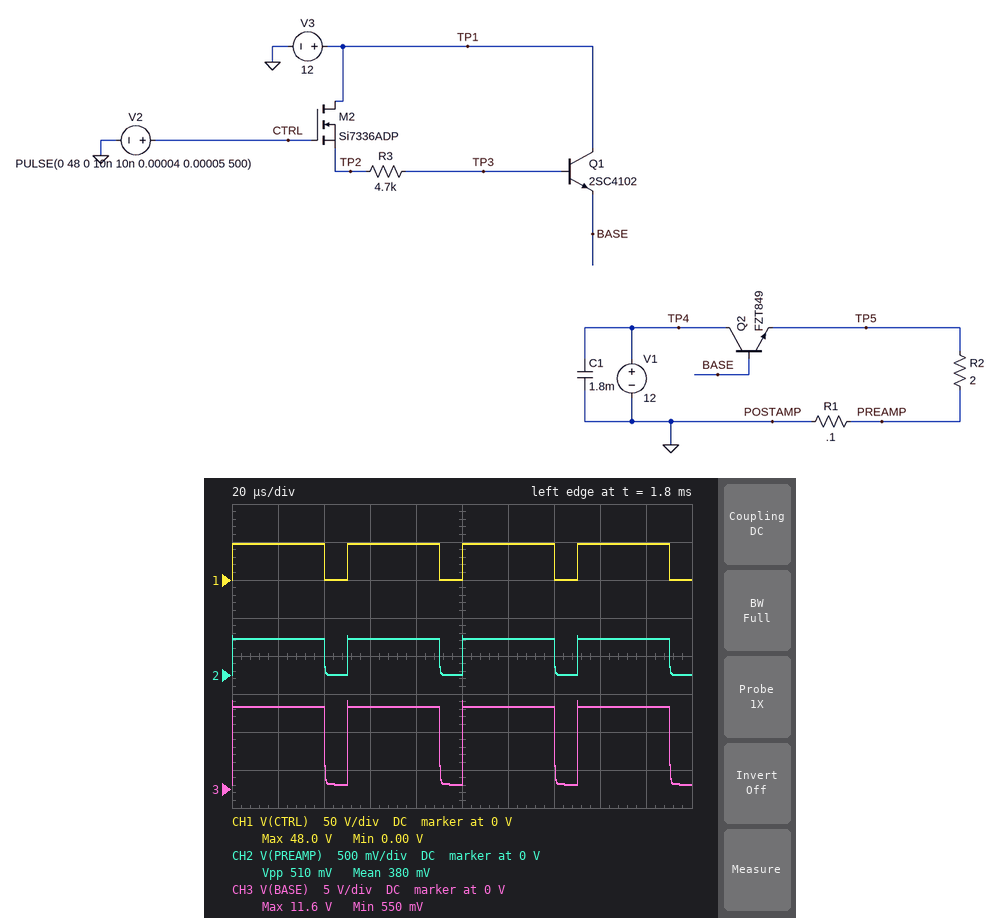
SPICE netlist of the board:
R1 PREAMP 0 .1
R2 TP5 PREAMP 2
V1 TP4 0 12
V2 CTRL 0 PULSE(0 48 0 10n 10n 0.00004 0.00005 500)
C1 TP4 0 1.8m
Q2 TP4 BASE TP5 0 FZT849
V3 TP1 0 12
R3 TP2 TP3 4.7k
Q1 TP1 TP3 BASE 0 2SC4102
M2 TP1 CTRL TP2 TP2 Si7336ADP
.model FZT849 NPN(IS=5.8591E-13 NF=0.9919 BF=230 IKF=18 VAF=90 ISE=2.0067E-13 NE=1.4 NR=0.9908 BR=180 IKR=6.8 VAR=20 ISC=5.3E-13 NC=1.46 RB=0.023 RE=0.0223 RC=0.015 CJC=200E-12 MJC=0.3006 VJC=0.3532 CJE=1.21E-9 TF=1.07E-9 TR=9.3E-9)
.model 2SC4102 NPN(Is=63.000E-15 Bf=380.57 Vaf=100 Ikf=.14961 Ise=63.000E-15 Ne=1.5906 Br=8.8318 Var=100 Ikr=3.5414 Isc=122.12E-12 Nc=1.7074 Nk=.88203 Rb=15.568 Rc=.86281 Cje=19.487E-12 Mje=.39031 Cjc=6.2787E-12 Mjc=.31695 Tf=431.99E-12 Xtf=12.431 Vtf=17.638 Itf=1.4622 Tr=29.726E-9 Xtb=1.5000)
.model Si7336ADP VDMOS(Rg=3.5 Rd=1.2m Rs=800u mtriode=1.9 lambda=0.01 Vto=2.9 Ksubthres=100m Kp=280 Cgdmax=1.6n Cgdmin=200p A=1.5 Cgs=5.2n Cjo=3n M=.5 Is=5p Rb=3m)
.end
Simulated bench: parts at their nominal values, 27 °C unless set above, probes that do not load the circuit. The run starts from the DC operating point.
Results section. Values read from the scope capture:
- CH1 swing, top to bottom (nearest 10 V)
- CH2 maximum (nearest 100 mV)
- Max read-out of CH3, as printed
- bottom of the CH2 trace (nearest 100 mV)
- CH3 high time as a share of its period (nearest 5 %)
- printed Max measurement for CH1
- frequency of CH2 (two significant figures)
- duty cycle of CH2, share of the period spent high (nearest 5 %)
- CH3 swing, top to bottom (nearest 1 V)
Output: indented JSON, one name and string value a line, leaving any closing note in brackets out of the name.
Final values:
{
  "CH1 swing, top to bottom": "50 V",
  "CH2 maximum": "500 mV",
  "Max read-out of CH3, as printed": "11.6 V",
  "bottom of the CH2 trace": "0 V",
  "CH3 high time as a share of its period": "80 %",
  "printed Max measurement for CH1": "48.0 V",
  "frequency of CH2": "20 kHz",
  "duty cycle of CH2, share of the period spent high": "80 %",
  "CH3 swing, top to bottom": "11 V"
}
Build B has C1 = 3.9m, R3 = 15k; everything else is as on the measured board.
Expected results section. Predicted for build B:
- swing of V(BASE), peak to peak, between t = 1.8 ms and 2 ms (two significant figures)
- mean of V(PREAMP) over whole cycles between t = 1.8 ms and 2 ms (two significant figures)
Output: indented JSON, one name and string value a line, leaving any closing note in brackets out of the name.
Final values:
{
  "swing of V(BASE), peak to peak, between t = 1.8 ms and 2 ms": "9.5 V",
  "mean of V(PREAMP) over whole cycles between t = 1.8 ms and 2 ms": "350 mV"
}
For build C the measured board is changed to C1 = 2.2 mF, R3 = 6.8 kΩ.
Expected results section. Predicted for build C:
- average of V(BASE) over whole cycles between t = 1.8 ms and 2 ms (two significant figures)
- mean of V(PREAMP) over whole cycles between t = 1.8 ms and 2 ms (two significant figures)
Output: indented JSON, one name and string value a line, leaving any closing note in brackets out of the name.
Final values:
{
  "average of V(BASE) over whole cycles between t = 1.8 ms and 2 ms": "8.7 V",
  "mean of V(PREAMP) over whole cycles between t = 1.8 ms and 2 ms": "370 mV"
}
